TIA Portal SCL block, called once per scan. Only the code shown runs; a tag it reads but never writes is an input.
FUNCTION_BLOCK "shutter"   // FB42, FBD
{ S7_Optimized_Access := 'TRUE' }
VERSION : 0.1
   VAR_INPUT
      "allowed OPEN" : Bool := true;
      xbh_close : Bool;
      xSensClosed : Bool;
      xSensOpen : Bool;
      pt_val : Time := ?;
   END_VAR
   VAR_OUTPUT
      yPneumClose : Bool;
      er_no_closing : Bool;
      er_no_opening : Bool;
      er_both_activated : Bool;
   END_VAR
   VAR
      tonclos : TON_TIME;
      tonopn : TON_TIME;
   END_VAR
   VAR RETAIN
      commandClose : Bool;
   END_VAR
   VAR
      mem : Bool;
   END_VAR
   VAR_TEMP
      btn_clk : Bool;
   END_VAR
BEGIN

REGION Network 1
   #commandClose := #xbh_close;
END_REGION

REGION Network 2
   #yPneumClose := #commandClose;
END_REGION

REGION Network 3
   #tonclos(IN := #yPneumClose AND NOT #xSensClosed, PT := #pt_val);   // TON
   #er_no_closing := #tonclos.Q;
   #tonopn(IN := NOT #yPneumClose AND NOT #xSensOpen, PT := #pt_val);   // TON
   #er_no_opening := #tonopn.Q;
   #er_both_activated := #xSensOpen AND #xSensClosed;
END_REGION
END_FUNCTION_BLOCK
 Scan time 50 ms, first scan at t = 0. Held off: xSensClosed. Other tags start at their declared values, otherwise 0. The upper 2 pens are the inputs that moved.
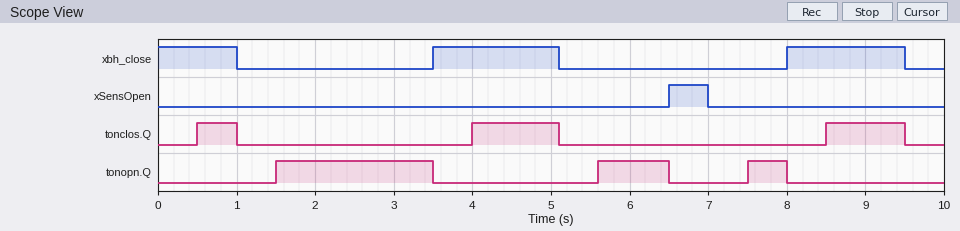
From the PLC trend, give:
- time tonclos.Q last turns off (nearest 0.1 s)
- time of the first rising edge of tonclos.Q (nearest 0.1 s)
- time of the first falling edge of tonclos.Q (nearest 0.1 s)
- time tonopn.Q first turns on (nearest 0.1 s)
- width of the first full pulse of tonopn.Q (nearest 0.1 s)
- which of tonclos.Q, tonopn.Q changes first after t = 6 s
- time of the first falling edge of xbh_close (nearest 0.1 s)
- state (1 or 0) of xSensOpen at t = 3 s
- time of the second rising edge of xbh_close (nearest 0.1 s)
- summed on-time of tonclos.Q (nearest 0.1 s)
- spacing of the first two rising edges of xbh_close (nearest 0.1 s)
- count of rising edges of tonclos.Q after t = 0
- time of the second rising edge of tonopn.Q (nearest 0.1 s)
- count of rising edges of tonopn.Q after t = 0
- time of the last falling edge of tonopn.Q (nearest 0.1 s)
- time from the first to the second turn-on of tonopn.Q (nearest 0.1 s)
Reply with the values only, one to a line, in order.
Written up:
9.5 s
0.5 s
1.0 s
1.5 s
2.0 s
tonopn.Q
1.0 s
0
8.0 s
2.6 s
4.5 s
3
5.6 s
3
8.0 s
4.1 s
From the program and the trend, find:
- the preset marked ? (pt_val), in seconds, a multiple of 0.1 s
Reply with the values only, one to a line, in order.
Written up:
0.5 s
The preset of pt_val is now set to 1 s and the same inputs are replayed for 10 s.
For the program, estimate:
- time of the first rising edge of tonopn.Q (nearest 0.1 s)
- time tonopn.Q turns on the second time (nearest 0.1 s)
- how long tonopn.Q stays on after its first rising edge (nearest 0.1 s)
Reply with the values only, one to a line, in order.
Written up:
2.0 s
6.1 s
1.5 s
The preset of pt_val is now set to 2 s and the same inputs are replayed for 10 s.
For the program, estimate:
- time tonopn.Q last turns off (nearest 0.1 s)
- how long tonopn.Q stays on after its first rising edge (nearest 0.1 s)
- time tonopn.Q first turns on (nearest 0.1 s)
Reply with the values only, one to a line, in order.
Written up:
3.5 s
0.5 s
3.0 s
